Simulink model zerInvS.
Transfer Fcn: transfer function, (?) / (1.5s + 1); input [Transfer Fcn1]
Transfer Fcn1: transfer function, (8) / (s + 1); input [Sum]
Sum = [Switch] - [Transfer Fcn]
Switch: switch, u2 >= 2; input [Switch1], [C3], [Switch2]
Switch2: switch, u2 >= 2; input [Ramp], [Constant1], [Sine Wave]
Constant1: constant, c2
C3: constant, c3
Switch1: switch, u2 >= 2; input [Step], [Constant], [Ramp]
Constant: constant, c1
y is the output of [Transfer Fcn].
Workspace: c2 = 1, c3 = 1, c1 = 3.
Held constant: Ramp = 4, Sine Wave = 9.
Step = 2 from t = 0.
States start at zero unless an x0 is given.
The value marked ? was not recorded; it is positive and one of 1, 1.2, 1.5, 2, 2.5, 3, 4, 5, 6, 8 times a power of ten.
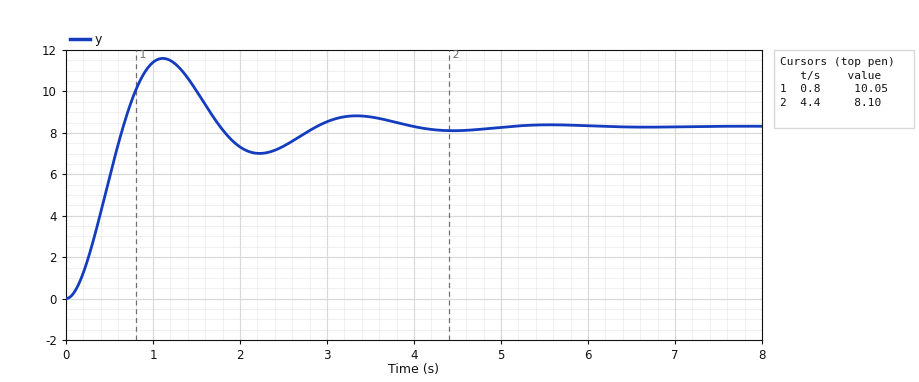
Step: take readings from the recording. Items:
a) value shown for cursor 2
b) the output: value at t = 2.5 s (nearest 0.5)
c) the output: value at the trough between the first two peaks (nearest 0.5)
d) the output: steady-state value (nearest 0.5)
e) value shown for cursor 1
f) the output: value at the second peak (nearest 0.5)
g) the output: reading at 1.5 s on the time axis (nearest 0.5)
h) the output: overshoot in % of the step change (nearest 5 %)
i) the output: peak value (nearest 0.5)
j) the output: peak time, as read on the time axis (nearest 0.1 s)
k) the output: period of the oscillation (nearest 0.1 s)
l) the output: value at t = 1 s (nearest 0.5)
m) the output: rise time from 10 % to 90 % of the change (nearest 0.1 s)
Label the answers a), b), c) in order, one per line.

a) 8.10
b) 7.5
c) 7.0
d) 8.5
e) 10.05
f) 9.0
g) 10.0
h) 40 %
i) 11.5
j) 1.1 s
k) 2.2 s
l) 11.5
m) 0.4 s
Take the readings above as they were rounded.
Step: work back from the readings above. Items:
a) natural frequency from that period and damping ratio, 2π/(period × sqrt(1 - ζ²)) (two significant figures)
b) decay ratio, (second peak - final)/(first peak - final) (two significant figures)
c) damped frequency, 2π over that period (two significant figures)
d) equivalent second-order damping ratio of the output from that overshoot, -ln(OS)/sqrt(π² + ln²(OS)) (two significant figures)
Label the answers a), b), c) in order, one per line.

a) 3.0 rad/s
b) 0.17
c) 2.9 rad/s
d) 0.28
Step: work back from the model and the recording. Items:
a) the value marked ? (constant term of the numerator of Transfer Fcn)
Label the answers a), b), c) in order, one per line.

a) 1.5
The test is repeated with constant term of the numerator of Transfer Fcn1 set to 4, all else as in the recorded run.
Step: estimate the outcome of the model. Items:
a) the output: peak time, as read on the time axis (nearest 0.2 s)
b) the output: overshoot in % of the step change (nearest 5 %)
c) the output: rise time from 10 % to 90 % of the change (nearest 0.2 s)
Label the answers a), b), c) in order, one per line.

a) 1.6 s
b) 25 %
c) 0.6 s
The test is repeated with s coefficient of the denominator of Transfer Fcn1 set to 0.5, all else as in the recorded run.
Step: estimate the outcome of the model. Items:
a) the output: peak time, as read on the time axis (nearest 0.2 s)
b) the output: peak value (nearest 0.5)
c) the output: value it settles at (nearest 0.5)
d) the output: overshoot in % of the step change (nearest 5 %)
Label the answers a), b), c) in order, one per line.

a) 0.8 s
b) 11.0
c) 8.5
d) 35 %
